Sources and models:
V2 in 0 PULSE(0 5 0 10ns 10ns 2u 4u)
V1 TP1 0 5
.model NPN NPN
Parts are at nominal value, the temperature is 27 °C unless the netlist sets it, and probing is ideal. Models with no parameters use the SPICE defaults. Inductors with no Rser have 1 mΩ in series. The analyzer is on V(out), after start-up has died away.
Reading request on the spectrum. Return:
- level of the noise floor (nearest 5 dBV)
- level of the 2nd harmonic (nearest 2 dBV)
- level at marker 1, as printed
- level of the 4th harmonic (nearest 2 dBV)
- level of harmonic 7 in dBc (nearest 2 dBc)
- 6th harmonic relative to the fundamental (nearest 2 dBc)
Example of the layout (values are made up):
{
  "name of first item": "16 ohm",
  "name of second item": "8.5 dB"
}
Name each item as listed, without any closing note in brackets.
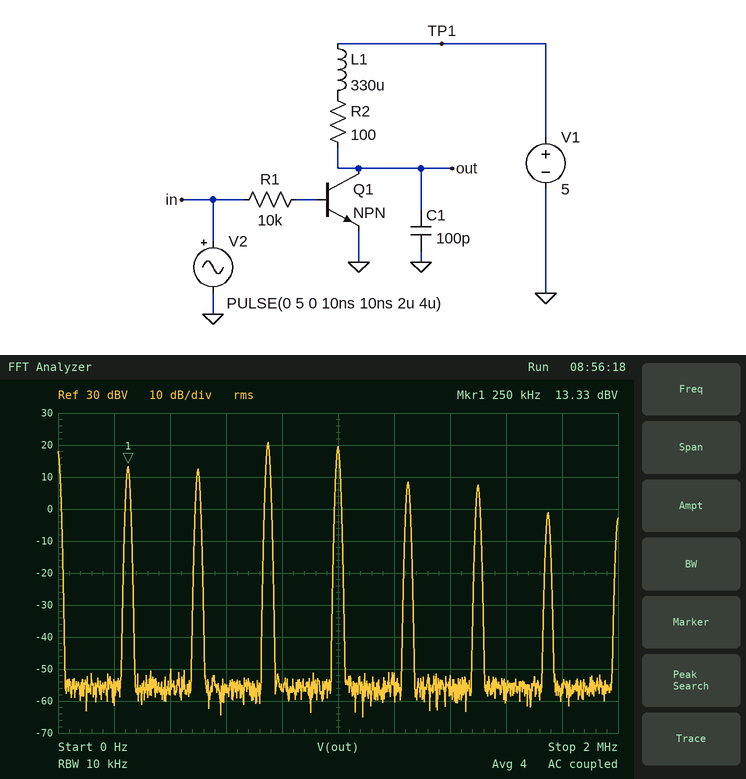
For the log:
{
  "level of the noise floor": "-55 dBV",
  "level of the 2nd harmonic": "12 dBV",
  "level at marker 1, as printed": "13.33 dBV",
  "level of the 4th harmonic": "20 dBV",
  "level of harmonic 7 in dBc": "-14 dBc",
  "6th harmonic relative to the fundamental": "-6 dBc"
}
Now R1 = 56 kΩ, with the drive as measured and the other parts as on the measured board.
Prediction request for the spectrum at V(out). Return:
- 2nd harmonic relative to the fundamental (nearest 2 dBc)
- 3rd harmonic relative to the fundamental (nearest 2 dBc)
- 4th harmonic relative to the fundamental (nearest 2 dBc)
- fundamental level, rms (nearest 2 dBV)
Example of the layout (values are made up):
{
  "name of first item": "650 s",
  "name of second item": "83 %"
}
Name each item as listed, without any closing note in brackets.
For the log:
{
  "2nd harmonic relative to the fundamental": "-8 dBc",
  "3rd harmonic relative to the fundamental": "10 dBc",
  "4th harmonic relative to the fundamental": "4 dBc",
  "fundamental level, rms": "6 dBV"
}
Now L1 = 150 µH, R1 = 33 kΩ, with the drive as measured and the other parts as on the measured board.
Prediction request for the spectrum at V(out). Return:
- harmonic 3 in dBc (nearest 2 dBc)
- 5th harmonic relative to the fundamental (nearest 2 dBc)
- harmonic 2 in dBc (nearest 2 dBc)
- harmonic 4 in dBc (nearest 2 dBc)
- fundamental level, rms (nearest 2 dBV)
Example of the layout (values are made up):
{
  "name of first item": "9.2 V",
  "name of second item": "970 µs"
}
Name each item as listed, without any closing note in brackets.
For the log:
{
  "harmonic 3 in dBc": "0 dBc",
  "5th harmonic relative to the fundamental": "8 dBc",
  "harmonic 2 in dBc": "-6 dBc",
  "harmonic 4 in dBc": "4 dBc",
  "fundamental level, rms": "4 dBV"
}
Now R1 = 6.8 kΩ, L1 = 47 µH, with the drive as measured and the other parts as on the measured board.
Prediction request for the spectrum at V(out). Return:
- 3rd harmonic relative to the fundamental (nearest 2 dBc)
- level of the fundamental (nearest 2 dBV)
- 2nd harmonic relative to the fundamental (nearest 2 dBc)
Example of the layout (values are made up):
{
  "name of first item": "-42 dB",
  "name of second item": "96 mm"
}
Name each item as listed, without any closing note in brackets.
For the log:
{
  "3rd harmonic relative to the fundamental": "-6 dBc",
  "level of the fundamental": "8 dBV",
  "2nd harmonic relative to the fundamental": "-8 dBc"
}
